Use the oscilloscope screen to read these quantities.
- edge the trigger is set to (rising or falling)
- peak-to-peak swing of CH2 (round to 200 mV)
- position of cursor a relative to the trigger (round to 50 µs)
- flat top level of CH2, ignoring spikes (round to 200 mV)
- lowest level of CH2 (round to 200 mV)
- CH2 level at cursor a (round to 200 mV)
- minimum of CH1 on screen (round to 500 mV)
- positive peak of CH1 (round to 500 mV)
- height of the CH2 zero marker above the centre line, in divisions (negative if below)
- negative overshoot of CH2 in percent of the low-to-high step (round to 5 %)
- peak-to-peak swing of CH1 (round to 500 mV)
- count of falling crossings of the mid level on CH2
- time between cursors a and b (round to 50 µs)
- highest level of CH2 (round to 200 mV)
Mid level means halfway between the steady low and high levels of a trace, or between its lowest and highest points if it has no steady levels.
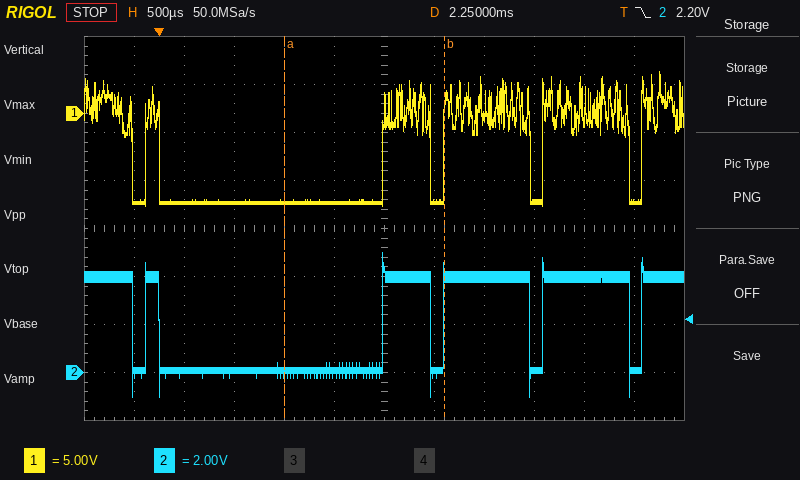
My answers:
falling
6.0 V
+1.25 ms
4.0 V
-1.0 V
0.0 V
-9.5 V
4.5 V
-3.0 div
30 %
14.0 V
5
1.60 ms
5.0 V
